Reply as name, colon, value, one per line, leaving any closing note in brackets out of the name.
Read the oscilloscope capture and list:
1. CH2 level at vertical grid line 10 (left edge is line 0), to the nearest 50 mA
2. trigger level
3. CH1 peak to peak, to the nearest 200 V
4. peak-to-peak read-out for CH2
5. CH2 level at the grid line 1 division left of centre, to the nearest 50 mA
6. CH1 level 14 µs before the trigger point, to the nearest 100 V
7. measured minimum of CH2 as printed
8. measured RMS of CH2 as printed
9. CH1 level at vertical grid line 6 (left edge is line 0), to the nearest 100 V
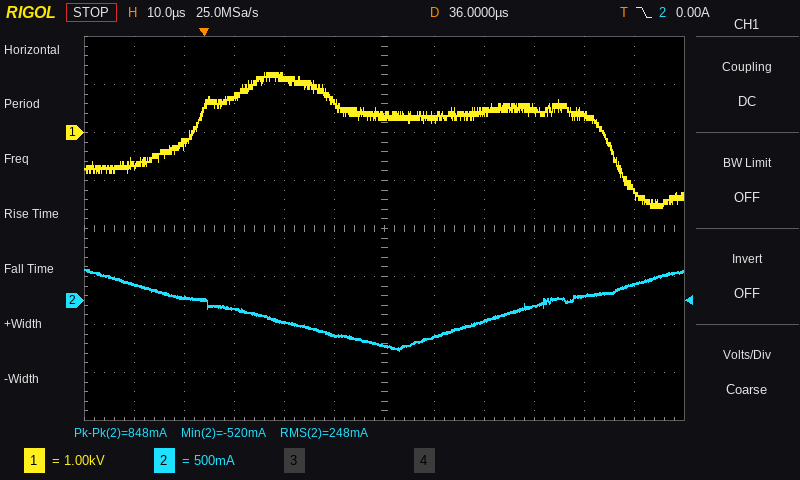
CH2 level at vertical grid line 10 (left edge is line 0), to the nearest 50 mA: 50 mA
trigger level: 0.00 A
CH1 peak to peak, to the nearest 200 V: 2.8 kV
peak-to-peak read-out for CH2: 848 mA
CH2 level at the grid line 1 division left of centre, to the nearest 50 mA: -350 mA
CH1 level 14 µs before the trigger point, to the nearest 100 V: -700 V
measured minimum of CH2 as printed: -520 mA
measured RMS of CH2 as printed: 248 mA
CH1 level at vertical grid line 6 (left edge is line 0), to the nearest 100 V: 400 V
